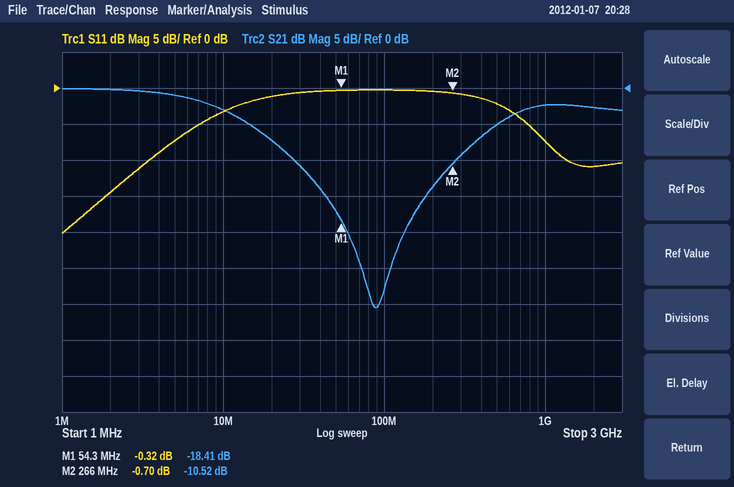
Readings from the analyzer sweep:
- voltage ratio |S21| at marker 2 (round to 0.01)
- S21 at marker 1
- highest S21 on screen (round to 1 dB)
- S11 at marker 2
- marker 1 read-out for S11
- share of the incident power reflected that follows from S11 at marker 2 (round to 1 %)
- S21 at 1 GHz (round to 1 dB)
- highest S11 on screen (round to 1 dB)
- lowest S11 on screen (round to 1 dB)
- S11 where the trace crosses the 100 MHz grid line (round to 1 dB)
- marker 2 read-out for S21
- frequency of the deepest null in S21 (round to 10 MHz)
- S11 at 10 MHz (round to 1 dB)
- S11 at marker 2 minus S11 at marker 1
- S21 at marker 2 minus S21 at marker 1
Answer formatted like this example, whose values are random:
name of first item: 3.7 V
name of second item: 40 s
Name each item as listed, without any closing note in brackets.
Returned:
voltage ratio |S21| at marker 2: 0.30
S21 at marker 1: -18.41 dB
highest S21 on screen: 0 dB
S11 at marker 2: -0.70 dB
marker 1 read-out for S11: -0.32 dB
share of the incident power reflected that follows from S11 at marker 2: 85 %
S21 at 1 GHz: -2 dB
highest S11 on screen: 0 dB
lowest S11 on screen: -20 dB
S11 where the trace crosses the 100 MHz grid line: 0 dB
marker 2 read-out for S21: -10.52 dB
frequency of the deepest null in S21: 90 MHz
S11 at 10 MHz: -3 dB
S11 at marker 2 minus S11 at marker 1: -0.38 dB
S21 at marker 2 minus S21 at marker 1: 7.89 dB
